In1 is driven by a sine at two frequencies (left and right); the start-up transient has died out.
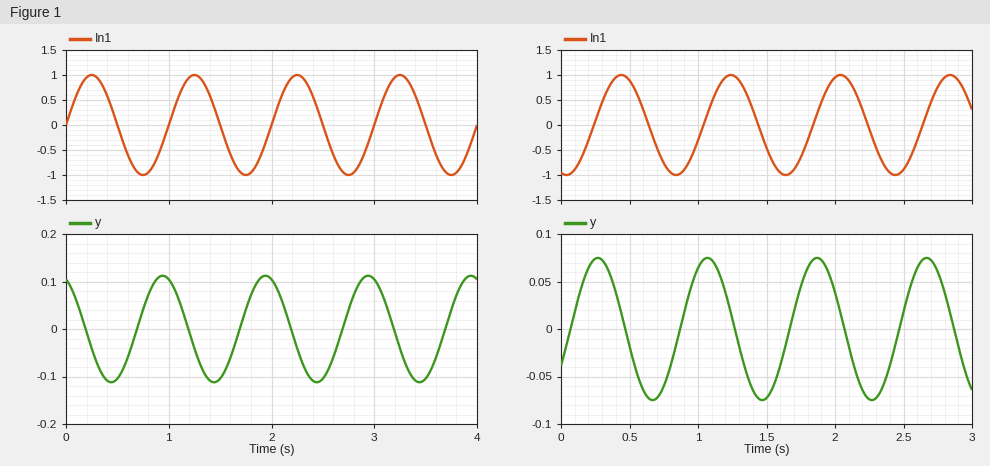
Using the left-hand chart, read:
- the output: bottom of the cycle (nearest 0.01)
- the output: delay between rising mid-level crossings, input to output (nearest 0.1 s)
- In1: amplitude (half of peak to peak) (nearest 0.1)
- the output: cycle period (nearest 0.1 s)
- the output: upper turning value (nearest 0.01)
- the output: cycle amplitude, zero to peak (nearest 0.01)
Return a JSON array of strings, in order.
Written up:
["-0.11", "0.7 s", "1.0", "1.0 s", "0.11", "0.11"]
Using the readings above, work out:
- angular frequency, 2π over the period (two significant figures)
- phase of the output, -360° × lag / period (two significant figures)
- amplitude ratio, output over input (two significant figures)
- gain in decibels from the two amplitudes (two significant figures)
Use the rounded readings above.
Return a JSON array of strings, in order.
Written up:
["6.3 rad/s", "-250°", "0.11", "-19 dB"]
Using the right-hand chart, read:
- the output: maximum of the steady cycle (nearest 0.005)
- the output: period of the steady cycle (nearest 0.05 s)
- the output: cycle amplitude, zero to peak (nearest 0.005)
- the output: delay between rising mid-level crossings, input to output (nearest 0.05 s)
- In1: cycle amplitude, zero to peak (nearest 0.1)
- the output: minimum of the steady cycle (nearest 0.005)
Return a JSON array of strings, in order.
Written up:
["0.075", "0.80 s", "0.075", "0.65 s", "1.0", "-0.075"]
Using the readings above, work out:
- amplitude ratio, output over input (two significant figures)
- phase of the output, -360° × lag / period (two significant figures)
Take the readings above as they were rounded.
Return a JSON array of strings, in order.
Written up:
["0.075", "-290°"]
